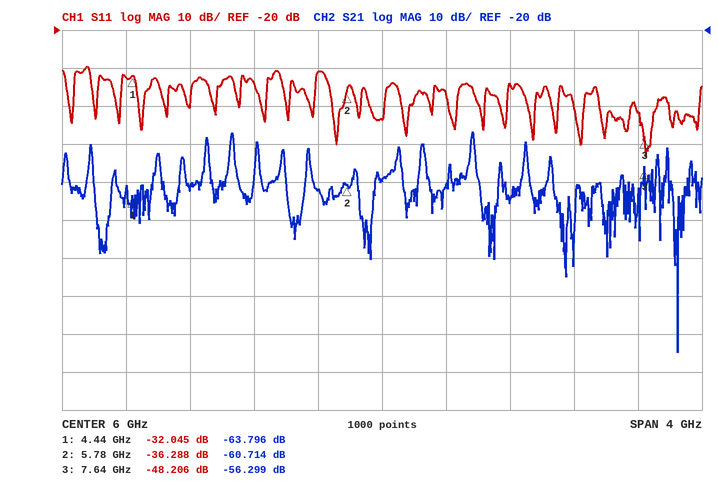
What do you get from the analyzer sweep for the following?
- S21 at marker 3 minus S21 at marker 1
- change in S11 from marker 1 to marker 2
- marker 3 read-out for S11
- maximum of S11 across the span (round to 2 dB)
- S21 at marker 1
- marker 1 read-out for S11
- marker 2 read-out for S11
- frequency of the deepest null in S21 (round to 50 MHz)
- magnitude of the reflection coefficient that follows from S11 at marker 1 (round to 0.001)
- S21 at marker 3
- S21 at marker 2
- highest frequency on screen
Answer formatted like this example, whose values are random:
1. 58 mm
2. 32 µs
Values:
1. 7.497 dB
2. -4.243 dB
3. -48.206 dB
4. -30 dB
5. -63.796 dB
6. -32.045 dB
7. -36.288 dB
8. 7.85 GHz
9. 0.025
10. -56.299 dB
11. -60.714 dB
12. 8 GHz
